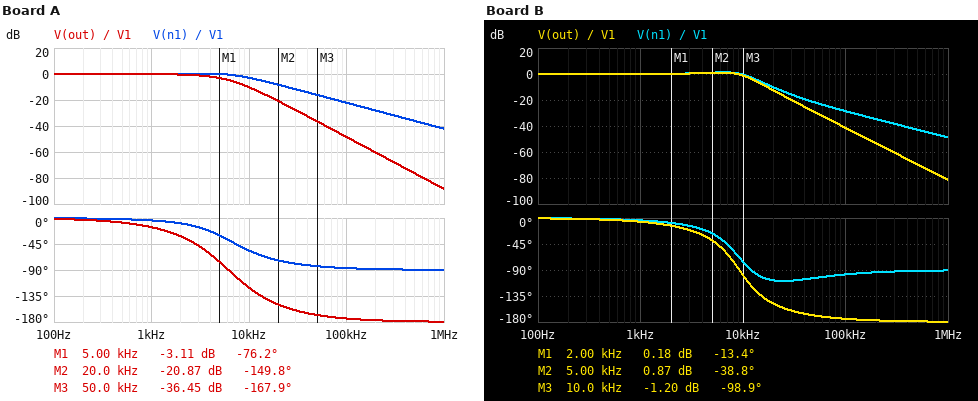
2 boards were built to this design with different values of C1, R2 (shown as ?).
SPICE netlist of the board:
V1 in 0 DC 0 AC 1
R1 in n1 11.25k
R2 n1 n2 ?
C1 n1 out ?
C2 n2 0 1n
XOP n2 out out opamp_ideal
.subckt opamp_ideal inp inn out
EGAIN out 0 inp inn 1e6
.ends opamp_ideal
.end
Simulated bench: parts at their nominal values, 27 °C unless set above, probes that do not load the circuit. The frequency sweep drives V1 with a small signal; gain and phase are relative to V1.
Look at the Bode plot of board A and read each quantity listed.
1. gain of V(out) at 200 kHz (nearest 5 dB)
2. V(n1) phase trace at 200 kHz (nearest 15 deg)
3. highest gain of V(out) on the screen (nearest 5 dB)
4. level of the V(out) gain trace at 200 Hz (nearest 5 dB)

-60 dB
-90 deg
0 dB
0 dB
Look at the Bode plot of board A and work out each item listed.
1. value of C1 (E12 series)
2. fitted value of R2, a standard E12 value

1.8 nF
33 kΩ
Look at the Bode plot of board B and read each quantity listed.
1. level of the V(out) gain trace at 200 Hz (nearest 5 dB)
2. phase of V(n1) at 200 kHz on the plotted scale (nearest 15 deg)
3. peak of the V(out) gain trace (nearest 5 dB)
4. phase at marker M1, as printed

0 dB
-90 deg
0 dB
-13.4 deg
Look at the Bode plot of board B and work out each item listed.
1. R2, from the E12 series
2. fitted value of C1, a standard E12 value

6.8 kΩ
3.9 nF
